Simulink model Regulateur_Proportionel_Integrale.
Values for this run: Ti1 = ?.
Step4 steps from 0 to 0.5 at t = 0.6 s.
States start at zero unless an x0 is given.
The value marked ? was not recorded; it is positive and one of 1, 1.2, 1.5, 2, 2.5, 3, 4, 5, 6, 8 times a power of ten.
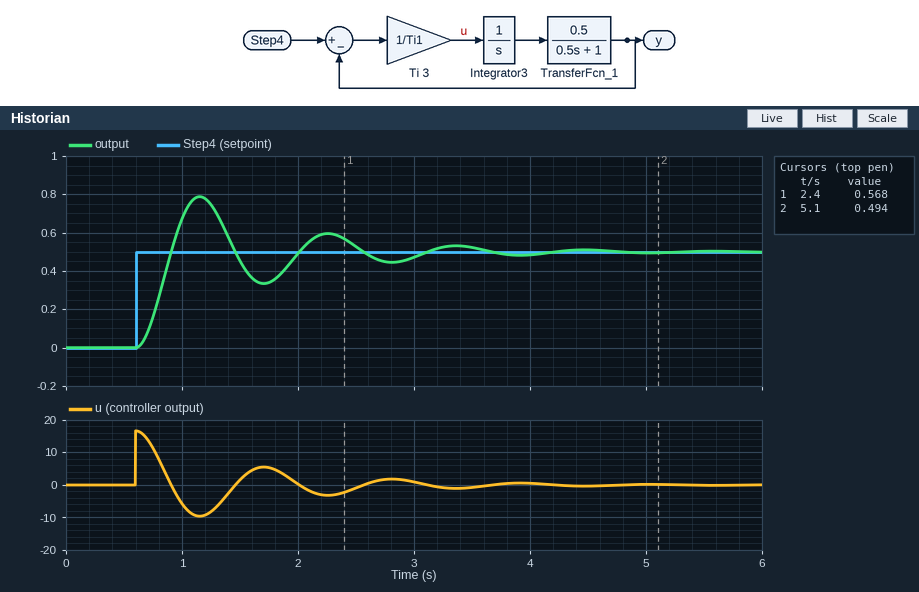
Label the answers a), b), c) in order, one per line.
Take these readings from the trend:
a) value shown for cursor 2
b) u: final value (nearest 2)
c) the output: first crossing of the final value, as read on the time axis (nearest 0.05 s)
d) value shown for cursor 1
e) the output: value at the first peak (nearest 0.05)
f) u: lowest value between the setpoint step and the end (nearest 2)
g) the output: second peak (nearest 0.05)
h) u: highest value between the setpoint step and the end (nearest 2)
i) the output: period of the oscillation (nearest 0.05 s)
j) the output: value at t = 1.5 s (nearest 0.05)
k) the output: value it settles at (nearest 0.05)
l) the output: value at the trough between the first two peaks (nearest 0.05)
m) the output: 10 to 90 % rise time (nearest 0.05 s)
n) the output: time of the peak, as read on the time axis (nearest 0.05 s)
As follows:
a) 0.494
b) 0
c) 0.90 s
d) 0.568
e) 0.80
f) -10
g) 0.60
h) 16
i) 1.10 s
j) 0.45
k) 0.50
l) 0.35
m) 0.20 s
n) 1.15 s
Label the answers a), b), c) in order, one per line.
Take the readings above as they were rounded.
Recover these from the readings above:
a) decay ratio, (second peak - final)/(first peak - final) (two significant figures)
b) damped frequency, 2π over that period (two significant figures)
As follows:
a) 0.33
b) 5.7 rad/s
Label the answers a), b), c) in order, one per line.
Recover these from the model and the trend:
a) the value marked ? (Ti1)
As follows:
a) 0.03
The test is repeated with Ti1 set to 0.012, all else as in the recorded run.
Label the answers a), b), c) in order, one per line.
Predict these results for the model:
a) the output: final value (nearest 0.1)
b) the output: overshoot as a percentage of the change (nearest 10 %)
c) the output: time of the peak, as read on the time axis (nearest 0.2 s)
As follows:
a) 0.5
b) 70 %
c) 1.0 s
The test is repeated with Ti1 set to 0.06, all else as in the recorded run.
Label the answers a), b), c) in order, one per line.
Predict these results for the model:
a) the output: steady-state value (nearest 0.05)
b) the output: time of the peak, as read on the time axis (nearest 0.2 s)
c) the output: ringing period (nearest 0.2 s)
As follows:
a) 0.50
b) 1.4 s
c) 1.6 s
